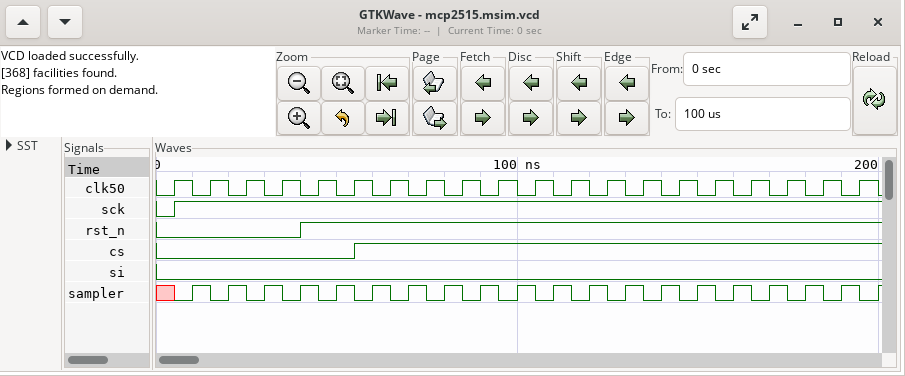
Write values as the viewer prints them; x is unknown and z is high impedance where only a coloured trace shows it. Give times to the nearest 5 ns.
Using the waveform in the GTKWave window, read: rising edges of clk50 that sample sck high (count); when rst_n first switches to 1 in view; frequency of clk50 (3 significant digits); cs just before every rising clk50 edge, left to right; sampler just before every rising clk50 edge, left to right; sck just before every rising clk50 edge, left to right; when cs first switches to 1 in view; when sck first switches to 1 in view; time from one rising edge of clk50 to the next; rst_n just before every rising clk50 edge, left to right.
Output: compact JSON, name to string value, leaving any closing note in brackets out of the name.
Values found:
{"rising edges of clk50 that sample sck high": "19", "when rst_n first switches to 1 in view": "40 ns", "frequency of clk50": "100 MHz", "cs just before every rising clk50 edge, left to right": "0 0 0 0 0 0 1 1 1 1 1 1 1 1 1 1 1 1 1 1", "sampler just before every rising clk50 edge, left to right": "x 1 1 1 1 1 1 1 1 1 1 1 1 1 1 1 1 1 1 1", "sck just before every rising clk50 edge, left to right": "0 1 1 1 1 1 1 1 1 1 1 1 1 1 1 1 1 1 1 1", "when cs first switches to 1 in view": "55 ns", "when sck first switches to 1 in view": "5 ns", "time from one rising edge of clk50 to the next": "10 ns", "rst_n just before every rising clk50 edge, left to right": "0 0 0 0 1 1 1 1 1 1 1 1 1 1 1 1 1 1 1 1"}
